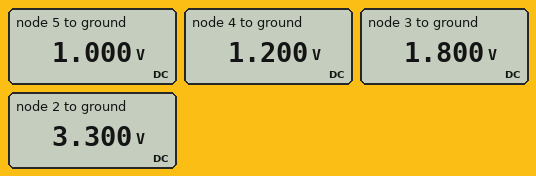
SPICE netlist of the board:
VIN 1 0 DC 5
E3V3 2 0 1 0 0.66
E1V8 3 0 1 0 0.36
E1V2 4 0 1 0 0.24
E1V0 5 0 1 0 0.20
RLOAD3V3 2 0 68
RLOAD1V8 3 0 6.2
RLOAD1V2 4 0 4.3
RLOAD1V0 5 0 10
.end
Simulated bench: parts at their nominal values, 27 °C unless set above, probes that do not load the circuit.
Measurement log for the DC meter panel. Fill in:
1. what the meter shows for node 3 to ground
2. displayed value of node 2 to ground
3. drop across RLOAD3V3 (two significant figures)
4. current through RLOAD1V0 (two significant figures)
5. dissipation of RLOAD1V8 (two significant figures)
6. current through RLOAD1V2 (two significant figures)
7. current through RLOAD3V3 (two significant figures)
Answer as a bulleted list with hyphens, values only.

- 1.800 V
- 3.300 V
- 3.3 V
- 100 mA
- 520 mW
- 280 mA
- 49 mA
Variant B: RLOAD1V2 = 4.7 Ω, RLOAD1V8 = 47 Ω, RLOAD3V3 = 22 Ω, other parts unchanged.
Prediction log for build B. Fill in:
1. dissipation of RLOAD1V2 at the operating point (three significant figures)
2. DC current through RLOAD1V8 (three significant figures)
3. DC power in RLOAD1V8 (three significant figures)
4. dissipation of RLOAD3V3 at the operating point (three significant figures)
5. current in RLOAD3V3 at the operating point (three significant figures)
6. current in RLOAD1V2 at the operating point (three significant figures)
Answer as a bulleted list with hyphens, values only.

- 306 mW
- 38.3 mA
- 68.9 mW
- 495 mW
- 150 mA
- 255 mA
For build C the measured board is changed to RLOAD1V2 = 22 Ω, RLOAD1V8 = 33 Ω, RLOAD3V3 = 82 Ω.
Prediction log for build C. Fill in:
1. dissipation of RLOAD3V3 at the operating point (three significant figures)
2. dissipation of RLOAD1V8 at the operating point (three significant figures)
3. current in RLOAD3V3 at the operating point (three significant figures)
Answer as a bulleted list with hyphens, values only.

- 133 mW
- 98.2 mW
- 40.2 mA
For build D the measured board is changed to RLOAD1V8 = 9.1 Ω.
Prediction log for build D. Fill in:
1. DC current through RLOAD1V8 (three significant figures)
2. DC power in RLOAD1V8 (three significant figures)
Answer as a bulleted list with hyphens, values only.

- 198 mA
- 356 mW
